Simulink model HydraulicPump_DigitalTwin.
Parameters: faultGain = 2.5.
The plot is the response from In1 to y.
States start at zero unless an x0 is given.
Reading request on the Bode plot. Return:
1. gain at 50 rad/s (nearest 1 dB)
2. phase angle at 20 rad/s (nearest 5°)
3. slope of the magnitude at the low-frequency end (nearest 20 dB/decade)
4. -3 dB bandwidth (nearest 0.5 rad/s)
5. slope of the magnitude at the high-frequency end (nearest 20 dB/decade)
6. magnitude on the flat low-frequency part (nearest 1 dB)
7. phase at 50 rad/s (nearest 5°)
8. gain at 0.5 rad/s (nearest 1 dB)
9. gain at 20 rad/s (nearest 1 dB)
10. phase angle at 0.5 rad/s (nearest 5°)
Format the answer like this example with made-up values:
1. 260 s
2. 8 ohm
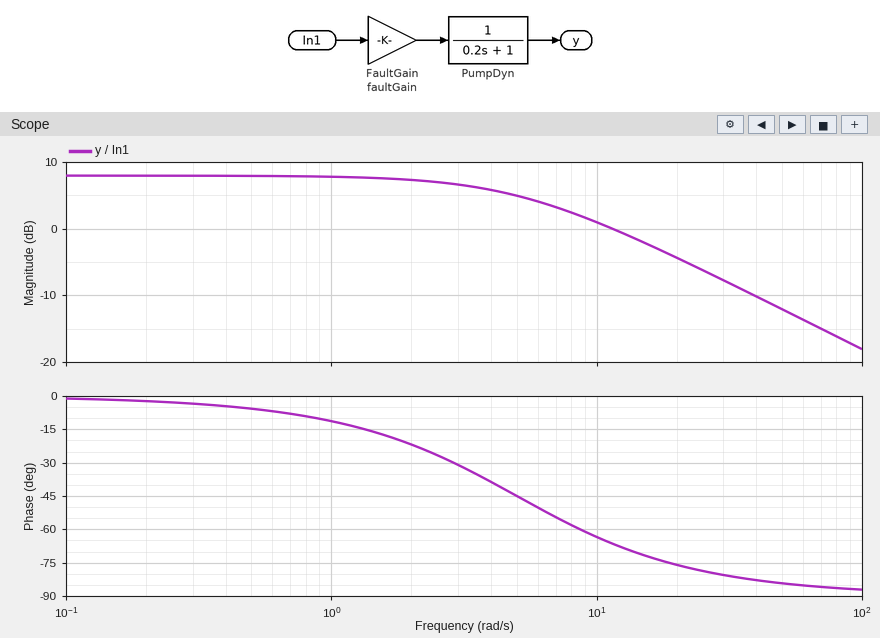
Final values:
1. -12 dB
2. -75°
3. 0 dB/decade
4. 5.0 rad/s
5. -20 dB/decade
6. 8 dB
7. -85°
8. 8 dB
9. -4 dB
10. -5°
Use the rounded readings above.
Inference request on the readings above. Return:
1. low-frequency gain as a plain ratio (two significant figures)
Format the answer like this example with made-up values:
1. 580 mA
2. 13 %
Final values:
1. 2.5
